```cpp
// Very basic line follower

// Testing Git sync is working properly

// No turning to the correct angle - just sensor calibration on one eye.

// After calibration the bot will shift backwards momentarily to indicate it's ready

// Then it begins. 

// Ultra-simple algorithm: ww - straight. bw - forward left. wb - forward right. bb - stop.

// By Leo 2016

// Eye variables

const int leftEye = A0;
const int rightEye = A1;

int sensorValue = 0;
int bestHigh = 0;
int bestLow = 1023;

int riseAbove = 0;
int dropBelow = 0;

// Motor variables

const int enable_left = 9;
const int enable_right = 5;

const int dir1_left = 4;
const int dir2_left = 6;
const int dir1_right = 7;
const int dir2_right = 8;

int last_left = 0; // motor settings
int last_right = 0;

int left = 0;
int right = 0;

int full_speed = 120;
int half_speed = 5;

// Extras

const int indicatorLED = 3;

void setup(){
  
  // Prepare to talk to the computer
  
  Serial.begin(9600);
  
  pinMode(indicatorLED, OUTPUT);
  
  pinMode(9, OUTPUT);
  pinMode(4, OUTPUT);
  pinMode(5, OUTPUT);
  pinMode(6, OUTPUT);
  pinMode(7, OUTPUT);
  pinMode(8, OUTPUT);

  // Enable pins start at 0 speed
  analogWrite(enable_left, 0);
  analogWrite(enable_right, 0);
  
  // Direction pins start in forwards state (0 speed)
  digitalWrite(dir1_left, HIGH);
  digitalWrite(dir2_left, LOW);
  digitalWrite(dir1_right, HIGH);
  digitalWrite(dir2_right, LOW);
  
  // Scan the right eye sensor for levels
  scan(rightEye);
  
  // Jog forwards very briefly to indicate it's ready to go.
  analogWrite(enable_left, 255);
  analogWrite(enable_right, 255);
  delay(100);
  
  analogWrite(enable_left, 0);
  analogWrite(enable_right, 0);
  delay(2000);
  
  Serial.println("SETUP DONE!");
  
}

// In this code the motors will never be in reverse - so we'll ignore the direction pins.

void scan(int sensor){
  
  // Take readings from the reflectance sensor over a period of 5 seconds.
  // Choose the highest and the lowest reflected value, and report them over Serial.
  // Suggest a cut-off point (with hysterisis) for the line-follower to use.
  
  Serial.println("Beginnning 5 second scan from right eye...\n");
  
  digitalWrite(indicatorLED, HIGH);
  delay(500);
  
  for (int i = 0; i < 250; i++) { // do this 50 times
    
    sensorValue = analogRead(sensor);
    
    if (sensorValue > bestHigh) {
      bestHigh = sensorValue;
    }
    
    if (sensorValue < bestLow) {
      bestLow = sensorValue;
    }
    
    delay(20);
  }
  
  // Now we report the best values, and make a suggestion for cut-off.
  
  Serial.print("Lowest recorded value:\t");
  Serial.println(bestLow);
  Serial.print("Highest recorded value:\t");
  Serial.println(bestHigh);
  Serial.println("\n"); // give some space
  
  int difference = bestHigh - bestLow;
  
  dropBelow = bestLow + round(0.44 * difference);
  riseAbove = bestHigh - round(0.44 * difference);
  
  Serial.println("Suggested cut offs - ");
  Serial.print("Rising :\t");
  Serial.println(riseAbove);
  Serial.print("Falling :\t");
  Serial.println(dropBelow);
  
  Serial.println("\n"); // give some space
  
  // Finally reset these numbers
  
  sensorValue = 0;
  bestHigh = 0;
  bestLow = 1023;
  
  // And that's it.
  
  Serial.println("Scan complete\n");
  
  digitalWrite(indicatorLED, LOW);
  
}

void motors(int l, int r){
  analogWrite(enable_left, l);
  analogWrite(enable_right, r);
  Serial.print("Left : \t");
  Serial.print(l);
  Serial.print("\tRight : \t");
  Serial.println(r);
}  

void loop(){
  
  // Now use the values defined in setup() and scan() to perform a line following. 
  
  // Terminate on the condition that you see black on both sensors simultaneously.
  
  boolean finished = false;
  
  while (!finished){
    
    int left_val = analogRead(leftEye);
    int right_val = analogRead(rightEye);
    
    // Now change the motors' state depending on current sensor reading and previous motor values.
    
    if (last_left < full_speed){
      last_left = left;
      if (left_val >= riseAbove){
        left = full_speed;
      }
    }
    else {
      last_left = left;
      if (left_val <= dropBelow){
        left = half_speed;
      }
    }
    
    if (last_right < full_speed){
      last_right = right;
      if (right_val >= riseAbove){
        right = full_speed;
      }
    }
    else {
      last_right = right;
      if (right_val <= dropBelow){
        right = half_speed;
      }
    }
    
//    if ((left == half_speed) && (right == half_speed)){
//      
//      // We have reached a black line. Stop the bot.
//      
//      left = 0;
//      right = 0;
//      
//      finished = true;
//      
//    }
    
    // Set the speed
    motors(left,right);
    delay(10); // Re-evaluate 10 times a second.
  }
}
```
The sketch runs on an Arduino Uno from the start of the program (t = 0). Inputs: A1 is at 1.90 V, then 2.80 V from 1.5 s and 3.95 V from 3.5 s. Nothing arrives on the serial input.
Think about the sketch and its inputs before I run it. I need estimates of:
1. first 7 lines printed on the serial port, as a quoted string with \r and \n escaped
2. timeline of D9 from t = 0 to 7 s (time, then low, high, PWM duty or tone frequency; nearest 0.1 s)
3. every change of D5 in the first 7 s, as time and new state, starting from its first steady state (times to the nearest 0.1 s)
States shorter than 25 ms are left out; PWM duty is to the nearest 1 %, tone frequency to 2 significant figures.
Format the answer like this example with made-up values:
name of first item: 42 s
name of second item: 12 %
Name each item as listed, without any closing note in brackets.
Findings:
first 7 lines printed on the serial port, as a quoted string with \r and \n escaped: "Beginnning 5 second scan from right eye...\n\r\nLowest recorded value:\t389\r\nHighest recorded value:\t808\r\n\n\r\nSuggested cut offs - \r\n"
timeline of D9 from t = 0 to 7 s: 0 s low; 5.6 s high; 5.7 s low
every change of D5 in the first 7 s, as time and new state, starting from its first steady state: 0 s low; 5.6 s high; 5.7 s low
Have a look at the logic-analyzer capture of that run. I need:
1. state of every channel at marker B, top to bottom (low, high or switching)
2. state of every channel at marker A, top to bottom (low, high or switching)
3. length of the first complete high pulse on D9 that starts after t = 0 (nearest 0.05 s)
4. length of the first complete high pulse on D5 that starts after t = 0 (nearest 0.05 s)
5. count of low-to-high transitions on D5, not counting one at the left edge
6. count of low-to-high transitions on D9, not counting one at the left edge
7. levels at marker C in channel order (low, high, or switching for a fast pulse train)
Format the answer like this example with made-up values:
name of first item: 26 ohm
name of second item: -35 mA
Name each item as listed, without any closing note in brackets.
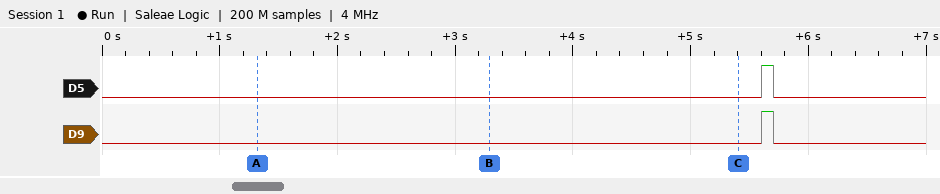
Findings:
state of every channel at marker B, top to bottom: D5 low, D9 low
state of every channel at marker A, top to bottom: D5 low, D9 low
length of the first complete high pulse on D9 that starts after t = 0: 0.10 s
length of the first complete high pulse on D5 that starts after t = 0: 0.10 s
count of low-to-high transitions on D5, not counting one at the left edge: 1
count of low-to-high transitions on D9, not counting one at the left edge: 1
levels at marker C in channel order: D5 low, D9 low
